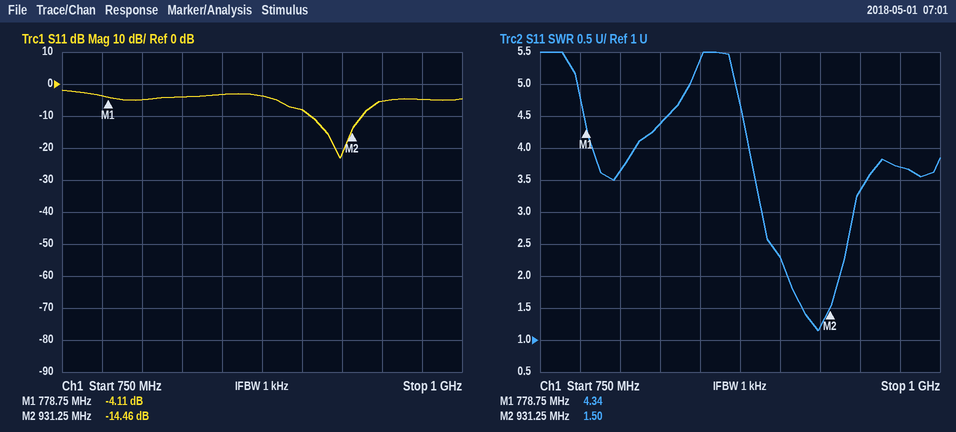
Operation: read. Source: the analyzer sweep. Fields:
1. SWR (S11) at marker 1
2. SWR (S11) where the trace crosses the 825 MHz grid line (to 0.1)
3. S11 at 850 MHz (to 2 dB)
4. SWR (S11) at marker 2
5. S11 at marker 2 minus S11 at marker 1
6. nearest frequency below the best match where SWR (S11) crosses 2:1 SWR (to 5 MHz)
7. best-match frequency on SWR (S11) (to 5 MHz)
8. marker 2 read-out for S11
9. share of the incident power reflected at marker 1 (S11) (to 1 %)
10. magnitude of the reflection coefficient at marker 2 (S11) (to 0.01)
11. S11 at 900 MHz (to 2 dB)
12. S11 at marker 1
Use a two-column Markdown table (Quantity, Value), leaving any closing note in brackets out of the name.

| Quantity | Value |
|---|---|
| SWR (S11) at marker 1 | 4.34 |
| SWR (S11) where the trace crosses the 825 MHz grid line | 4.4 |
| S11 at 850 MHz | -4 dB |
| SWR (S11) at marker 2 | 1.50 |
| S11 at marker 2 minus S11 at marker 1 | -10.35 dB |
| nearest frequency below the best match where SWR (S11) crosses 2:1 SWR | 905 MHz |
| best-match frequency on SWR (S11) | 925 MHz |
| marker 2 read-out for S11 | -14.46 dB |
| share of the incident power reflected at marker 1 (S11) | 39 % |
| magnitude of the reflection coefficient at marker 2 (S11) | 0.19 |
| S11 at 900 MHz | -8 dB |
| S11 at marker 1 | -4.11 dB |
